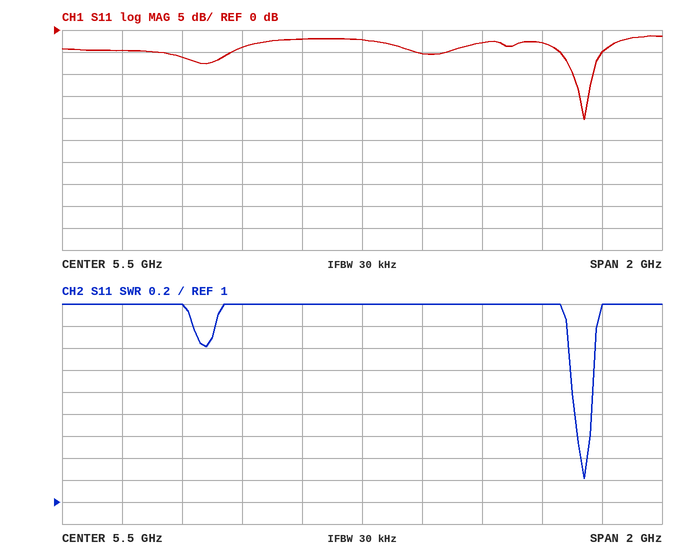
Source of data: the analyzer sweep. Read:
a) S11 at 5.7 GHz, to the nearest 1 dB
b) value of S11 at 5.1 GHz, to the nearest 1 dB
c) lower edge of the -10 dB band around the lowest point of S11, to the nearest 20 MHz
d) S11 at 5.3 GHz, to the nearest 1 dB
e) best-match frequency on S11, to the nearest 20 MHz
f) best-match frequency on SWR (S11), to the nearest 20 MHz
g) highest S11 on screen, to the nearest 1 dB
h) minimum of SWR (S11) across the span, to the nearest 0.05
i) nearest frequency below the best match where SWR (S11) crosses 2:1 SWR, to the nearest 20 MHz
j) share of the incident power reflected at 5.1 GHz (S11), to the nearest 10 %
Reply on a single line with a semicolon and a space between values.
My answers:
-5 dB; -4 dB; 6.20 GHz; -2 dB; 6.24 GHz; 6.24 GHz; -1 dB; 1.20; 6.20 GHz; 40 %
